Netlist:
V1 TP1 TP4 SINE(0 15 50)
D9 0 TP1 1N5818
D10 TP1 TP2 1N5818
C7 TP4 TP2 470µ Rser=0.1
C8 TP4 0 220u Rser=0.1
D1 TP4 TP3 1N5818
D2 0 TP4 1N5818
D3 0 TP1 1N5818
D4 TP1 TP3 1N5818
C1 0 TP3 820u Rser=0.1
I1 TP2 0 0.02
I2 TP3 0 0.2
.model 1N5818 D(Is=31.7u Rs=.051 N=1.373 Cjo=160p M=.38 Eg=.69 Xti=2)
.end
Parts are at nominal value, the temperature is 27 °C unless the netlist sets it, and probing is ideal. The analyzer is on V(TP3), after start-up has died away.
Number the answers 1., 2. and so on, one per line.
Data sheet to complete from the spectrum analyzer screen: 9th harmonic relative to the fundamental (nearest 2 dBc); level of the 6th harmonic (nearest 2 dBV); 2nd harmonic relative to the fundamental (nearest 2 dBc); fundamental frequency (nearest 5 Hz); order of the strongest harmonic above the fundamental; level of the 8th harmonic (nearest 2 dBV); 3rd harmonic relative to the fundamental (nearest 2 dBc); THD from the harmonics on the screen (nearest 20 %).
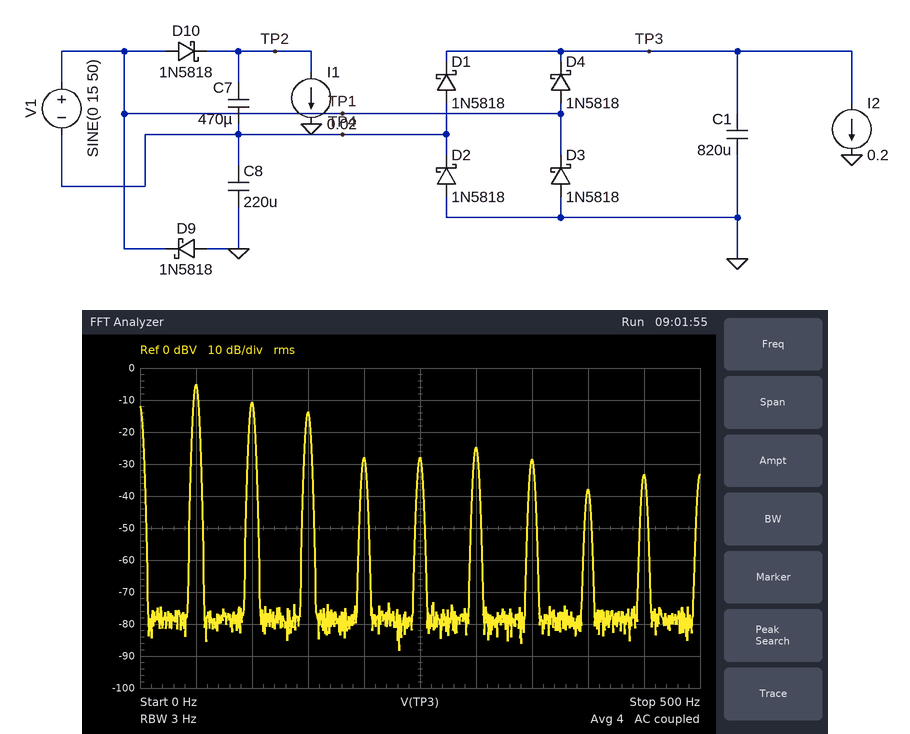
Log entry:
1. -28 dBc
2. -24 dBV
3. -6 dBc
4. 50 Hz
5. 2
6. -38 dBV
7. -8 dBc
8. 60 %
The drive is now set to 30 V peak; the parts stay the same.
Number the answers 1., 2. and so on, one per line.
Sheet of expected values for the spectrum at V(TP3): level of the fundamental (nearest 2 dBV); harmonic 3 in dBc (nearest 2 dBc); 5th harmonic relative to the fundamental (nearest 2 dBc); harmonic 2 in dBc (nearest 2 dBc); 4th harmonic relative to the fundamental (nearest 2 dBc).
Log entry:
1. 0 dBV
2. -14 dBc
3. -26 dBc
4. -8 dBc
5. -20 dBc
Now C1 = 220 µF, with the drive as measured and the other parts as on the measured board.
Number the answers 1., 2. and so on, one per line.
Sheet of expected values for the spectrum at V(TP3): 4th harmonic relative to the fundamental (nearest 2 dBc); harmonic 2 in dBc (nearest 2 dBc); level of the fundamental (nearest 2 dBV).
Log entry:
1. -20 dBc
2. -2 dBc
3. 2 dBV
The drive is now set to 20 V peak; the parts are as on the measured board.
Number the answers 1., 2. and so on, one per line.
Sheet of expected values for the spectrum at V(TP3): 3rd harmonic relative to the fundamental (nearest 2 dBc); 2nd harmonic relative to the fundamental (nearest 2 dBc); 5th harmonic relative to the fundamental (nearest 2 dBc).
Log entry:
1. -14 dBc
2. -8 dBc
3. -34 dBc
